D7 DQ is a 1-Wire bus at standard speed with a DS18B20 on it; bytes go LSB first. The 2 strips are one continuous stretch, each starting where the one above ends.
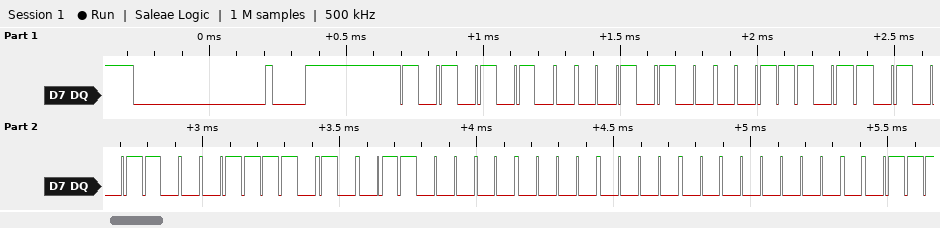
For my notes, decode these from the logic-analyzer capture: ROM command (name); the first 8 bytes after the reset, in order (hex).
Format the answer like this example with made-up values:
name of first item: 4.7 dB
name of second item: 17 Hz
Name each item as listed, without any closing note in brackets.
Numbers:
ROM command: Match ROM
the first 8 bytes after the reset, in order: 55 28 DC 32 5E 06 00 00
